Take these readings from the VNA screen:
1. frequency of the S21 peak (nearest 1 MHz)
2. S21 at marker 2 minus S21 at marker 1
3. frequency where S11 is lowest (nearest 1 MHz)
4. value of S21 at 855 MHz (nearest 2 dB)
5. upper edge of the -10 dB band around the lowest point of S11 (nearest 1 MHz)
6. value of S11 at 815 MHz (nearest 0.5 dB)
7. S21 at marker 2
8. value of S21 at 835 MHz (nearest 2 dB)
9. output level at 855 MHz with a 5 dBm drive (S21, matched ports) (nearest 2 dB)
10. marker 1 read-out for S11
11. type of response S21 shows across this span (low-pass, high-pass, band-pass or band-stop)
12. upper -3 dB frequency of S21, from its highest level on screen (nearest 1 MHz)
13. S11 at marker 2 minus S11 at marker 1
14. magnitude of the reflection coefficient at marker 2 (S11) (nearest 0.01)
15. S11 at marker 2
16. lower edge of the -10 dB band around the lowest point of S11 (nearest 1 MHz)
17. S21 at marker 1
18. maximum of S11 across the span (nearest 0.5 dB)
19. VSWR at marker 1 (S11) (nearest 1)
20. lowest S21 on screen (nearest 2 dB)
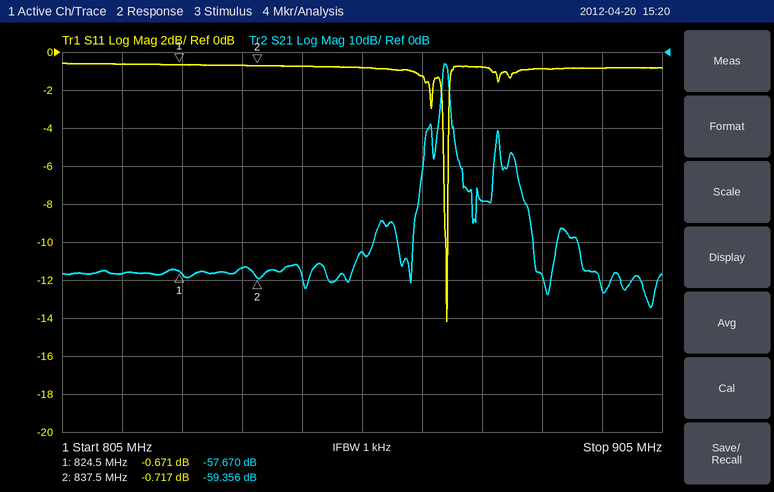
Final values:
869 MHz
-1.686 dB
869 MHz
-52 dB
869 MHz
-0.5 dB
-59.356 dB
-56 dB
-48 dBm
-0.671 dB
band-pass
869 MHz
-0.046 dB
0.92
-0.717 dB
869 MHz
-57.670 dB
-0.5 dB
26
-68 dB
